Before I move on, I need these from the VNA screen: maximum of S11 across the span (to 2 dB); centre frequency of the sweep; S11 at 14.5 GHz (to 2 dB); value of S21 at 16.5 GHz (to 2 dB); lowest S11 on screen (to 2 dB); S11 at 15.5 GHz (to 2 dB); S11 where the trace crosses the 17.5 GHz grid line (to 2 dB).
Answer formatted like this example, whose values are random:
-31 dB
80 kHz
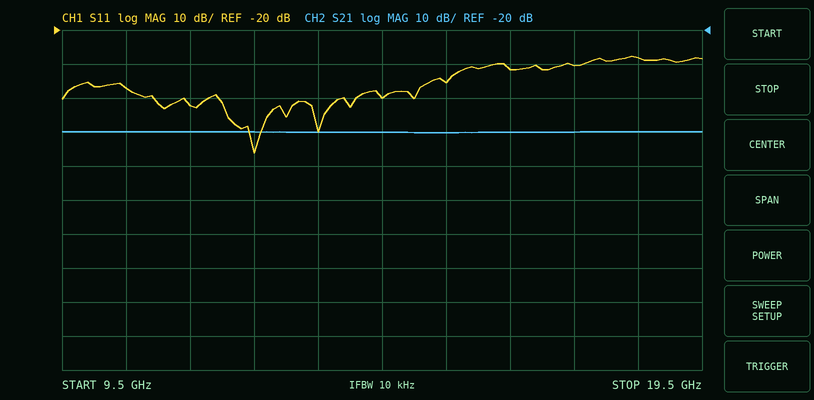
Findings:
-28 dB
14.5 GHz
-40 dB
-50 dB
-56 dB
-36 dB
-30 dB
